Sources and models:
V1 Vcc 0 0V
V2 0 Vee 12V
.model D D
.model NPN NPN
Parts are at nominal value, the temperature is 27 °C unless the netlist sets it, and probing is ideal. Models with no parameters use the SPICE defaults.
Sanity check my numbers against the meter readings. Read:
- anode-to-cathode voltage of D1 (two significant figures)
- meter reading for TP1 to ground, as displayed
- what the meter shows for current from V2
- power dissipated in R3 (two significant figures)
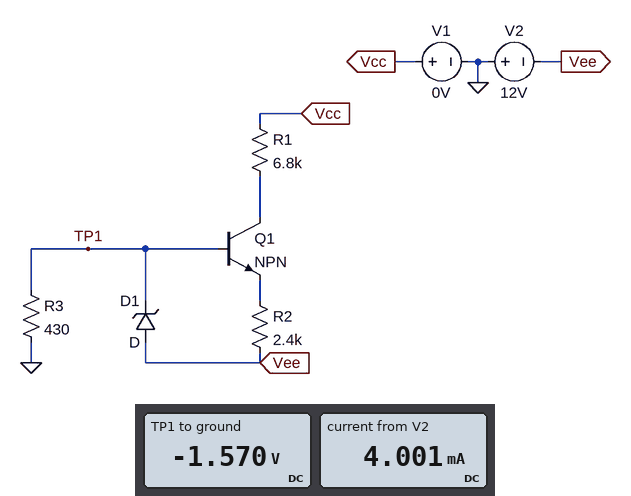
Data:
-10 V
-1.570 V
4.001 mA
5.7 mW
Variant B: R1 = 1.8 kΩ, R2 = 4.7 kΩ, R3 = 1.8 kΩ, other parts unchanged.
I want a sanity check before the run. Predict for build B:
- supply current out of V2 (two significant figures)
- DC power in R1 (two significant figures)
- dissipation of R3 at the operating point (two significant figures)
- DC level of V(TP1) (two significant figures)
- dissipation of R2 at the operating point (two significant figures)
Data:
2.1 mA
2.8 mW
1.2 mW
-1.5 V
20 mW
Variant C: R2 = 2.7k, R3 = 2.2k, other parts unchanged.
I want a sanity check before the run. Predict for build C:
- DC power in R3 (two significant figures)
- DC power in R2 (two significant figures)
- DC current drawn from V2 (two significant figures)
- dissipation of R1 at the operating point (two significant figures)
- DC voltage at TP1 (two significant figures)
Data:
7.8 mW
18 mW
2.6 mA
3.6 mW
-4.1 V
